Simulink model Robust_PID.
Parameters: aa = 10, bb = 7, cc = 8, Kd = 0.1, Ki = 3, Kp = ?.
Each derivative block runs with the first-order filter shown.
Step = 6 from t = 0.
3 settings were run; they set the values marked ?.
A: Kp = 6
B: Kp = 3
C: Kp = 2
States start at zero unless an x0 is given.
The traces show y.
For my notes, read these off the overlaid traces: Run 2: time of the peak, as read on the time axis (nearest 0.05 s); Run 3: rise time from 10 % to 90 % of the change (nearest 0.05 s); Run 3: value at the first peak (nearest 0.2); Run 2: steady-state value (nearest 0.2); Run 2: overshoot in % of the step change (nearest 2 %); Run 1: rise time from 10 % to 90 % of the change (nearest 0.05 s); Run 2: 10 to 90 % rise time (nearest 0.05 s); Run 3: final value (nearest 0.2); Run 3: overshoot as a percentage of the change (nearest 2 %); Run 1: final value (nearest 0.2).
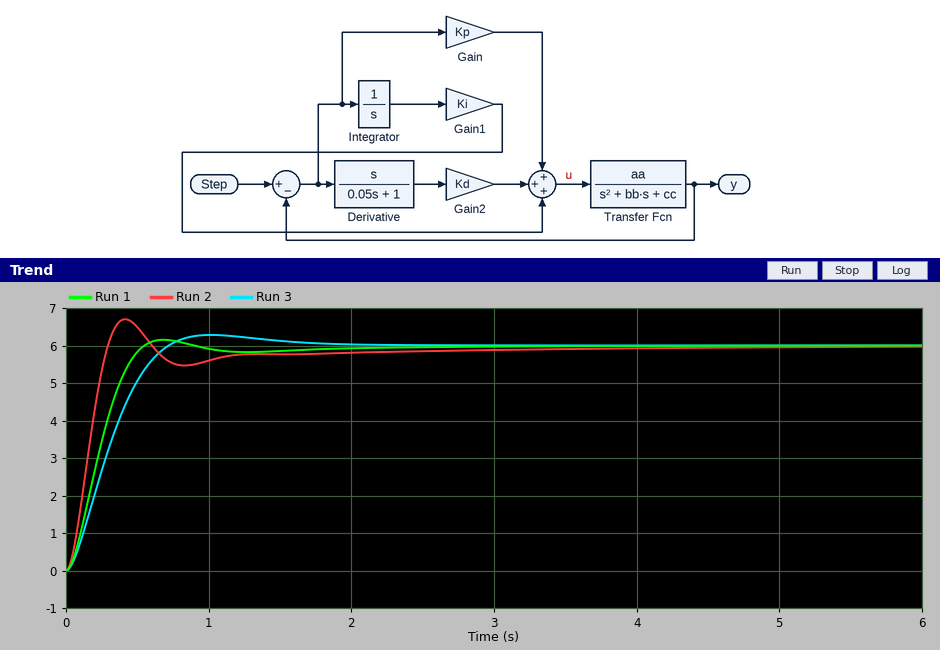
0.40 s
0.45 s
6.2
6.0
12 %
0.35 s
0.20 s
6.0
4 %
6.0
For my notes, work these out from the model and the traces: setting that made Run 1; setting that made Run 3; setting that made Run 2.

B
C
A
